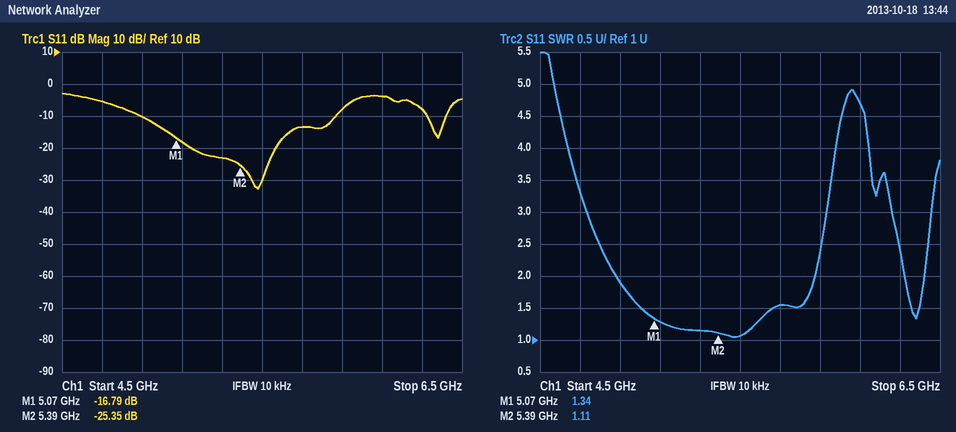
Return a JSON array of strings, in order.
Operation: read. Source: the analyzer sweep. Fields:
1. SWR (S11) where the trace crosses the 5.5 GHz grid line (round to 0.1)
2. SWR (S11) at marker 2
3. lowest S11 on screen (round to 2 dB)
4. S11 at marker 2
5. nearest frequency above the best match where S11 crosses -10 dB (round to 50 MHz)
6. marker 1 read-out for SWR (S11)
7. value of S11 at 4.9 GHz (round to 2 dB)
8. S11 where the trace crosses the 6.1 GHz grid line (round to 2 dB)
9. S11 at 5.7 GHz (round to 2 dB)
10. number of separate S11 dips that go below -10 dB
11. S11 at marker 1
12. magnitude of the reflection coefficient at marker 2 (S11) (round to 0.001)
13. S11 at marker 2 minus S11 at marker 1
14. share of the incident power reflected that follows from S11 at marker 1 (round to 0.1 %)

["1.1", "1.11", "-32 dB", "-25.35 dB", "5.85 GHz", "1.34", "-10 dB", "-4 dB", "-14 dB", "2", "-16.79 dB", "0.054", "-8.56 dB", "2.1 %"]
